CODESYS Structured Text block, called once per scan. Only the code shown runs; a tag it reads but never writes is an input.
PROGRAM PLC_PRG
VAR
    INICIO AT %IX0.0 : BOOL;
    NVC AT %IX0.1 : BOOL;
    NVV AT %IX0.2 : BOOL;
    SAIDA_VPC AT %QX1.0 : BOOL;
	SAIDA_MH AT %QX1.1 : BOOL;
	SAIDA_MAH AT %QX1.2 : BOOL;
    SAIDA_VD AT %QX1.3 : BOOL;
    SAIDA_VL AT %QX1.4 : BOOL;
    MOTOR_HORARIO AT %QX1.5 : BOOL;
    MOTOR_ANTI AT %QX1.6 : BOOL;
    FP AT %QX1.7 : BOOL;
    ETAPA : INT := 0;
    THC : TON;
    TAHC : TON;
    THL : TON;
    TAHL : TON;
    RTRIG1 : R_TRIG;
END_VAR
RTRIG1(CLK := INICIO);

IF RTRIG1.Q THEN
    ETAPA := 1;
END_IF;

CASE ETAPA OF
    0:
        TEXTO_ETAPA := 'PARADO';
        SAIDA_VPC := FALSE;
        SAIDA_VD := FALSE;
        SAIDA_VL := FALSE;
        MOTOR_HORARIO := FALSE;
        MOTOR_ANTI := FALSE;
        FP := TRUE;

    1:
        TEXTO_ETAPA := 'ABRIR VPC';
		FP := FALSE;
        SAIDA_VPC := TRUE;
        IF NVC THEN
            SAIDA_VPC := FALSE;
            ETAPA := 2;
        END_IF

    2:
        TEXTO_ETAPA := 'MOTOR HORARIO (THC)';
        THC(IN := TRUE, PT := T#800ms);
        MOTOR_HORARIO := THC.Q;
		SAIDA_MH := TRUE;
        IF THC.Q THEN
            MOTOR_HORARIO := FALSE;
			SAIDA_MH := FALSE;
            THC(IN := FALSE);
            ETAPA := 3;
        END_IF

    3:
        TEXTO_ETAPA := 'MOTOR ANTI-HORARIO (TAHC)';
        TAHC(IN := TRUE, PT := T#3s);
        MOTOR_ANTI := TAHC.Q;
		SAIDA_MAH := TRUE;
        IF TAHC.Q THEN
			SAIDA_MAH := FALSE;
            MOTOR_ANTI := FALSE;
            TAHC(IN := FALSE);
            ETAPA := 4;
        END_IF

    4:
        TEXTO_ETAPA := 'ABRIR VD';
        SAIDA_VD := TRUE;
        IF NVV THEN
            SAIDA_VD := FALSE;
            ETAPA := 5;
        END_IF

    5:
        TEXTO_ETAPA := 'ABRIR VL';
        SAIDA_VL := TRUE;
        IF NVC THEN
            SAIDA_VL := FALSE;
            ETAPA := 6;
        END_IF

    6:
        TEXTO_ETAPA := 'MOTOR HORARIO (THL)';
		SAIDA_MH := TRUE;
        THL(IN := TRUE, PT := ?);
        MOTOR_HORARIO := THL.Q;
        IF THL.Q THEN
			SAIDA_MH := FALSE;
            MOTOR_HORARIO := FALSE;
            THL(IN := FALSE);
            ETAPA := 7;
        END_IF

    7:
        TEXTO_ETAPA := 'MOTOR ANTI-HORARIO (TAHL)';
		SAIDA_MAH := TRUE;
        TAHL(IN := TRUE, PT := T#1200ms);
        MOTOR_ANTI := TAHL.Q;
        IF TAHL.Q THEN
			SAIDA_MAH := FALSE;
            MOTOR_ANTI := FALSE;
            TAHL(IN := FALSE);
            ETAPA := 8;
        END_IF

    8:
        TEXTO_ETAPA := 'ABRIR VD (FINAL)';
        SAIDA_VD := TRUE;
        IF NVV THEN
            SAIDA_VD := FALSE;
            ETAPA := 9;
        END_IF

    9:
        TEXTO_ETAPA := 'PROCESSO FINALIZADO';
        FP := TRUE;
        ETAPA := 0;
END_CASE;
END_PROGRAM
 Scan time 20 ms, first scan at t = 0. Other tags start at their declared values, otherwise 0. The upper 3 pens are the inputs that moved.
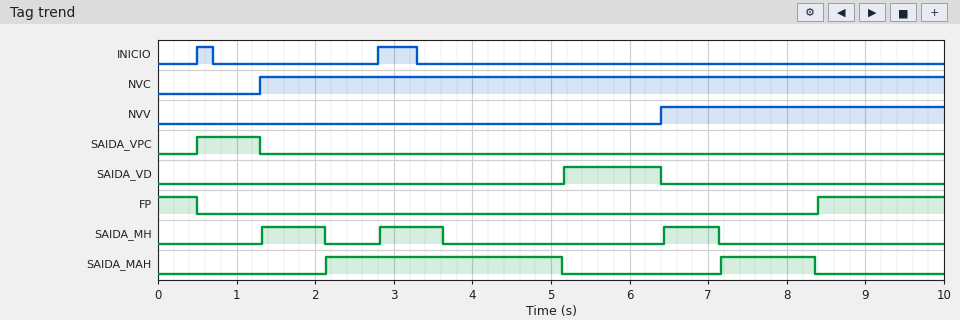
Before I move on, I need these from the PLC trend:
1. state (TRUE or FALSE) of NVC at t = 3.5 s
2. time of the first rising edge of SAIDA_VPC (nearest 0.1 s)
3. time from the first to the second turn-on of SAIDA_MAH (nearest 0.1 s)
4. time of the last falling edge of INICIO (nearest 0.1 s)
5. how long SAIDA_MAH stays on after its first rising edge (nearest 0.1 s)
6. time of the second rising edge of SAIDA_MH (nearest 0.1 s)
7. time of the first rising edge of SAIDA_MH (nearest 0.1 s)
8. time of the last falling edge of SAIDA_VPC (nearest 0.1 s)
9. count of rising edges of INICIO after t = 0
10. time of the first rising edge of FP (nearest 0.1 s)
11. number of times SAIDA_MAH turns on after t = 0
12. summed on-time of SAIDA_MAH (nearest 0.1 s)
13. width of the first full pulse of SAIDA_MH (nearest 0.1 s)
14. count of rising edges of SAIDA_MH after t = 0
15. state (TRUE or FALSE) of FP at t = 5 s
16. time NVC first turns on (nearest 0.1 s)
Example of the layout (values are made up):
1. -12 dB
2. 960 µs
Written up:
1. TRUE
2. 0.5 s
3. 5.0 s
4. 3.3 s
5. 3.0 s
6. 2.8 s
7. 1.3 s
8. 1.3 s
9. 2
10. 8.4 s
11. 2
12. 4.2 s
13. 0.8 s
14. 3
15. FALSE
16. 1.3 s
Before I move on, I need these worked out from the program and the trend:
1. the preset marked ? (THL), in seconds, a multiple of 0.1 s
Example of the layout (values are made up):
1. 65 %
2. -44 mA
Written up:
1. 0.7 s
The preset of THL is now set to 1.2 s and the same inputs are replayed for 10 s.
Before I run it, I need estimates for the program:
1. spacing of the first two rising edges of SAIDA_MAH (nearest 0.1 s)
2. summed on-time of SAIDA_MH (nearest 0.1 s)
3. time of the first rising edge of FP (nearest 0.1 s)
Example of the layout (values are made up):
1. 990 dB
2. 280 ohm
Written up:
1. 5.5 s
2. 2.8 s
3. 8.9 s
